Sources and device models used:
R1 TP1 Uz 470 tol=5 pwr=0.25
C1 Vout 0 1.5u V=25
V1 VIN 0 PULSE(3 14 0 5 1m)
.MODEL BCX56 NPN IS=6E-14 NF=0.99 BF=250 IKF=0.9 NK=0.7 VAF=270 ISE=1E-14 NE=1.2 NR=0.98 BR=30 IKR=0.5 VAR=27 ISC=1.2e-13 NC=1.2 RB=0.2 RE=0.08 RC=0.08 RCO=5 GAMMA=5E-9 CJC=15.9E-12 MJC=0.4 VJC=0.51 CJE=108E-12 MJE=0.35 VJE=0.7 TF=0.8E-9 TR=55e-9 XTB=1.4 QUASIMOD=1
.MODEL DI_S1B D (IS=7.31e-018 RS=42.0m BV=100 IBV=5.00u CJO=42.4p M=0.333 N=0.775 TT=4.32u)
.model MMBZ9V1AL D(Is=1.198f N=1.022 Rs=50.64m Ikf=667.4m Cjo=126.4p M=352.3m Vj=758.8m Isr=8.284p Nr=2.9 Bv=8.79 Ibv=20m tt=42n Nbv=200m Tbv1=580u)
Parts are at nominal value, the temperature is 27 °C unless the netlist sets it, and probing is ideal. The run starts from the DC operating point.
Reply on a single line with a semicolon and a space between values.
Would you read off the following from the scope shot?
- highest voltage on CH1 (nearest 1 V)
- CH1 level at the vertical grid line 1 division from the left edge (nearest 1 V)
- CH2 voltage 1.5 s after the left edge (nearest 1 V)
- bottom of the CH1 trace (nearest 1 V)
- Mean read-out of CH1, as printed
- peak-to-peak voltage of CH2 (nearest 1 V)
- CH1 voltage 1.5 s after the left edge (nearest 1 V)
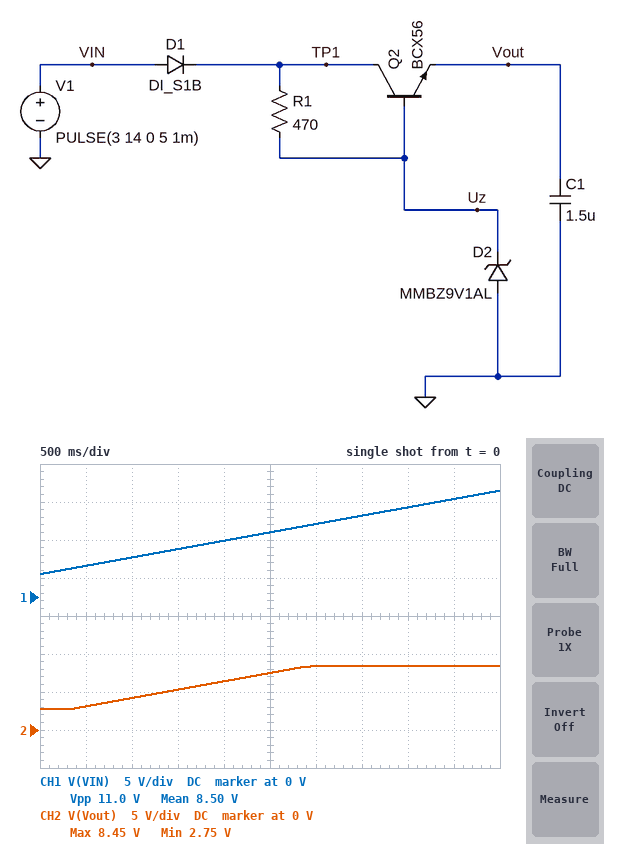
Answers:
14 V; 4 V; 5 V; 3 V; 8.50 V; 6 V; 6 V
